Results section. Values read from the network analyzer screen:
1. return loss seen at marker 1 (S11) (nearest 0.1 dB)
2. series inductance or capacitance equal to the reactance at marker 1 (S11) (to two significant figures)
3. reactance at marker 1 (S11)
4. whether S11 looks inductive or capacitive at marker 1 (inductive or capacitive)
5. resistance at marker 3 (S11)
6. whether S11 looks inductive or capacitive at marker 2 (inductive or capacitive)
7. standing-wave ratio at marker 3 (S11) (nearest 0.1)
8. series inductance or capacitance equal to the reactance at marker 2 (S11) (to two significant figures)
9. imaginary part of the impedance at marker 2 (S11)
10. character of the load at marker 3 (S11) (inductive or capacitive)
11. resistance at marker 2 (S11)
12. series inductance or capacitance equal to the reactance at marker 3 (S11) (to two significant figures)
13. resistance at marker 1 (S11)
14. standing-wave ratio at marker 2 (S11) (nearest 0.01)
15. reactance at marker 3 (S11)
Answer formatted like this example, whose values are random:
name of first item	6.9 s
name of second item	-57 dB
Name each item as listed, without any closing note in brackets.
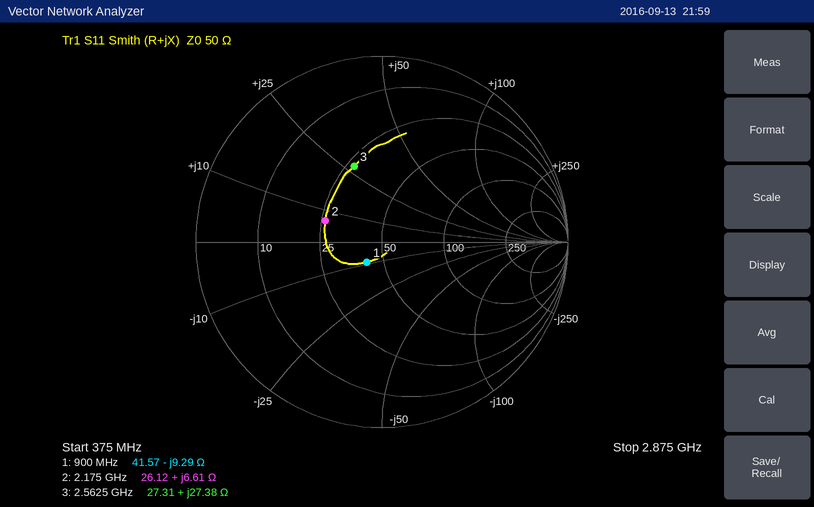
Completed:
return loss seen at marker 1 (S11)	17.3 dB
series inductance or capacitance equal to the reactance at marker 1 (S11)	19 pF
reactance at marker 1	-9.29 Ω
whether S11 looks inductive or capacitive at marker 1	capacitive
resistance at marker 3	27.31 Ω
whether S11 looks inductive or capacitive at marker 2	inductive
standing-wave ratio at marker 3 (S11)	2.5
series inductance or capacitance equal to the reactance at marker 2 (S11)	480 pH
imaginary part of the impedance at marker 2	+6.61 Ω
character of the load at marker 3 (S11)	inductive
resistance at marker 2	26.12 Ω
series inductance or capacitance equal to the reactance at marker 3 (S11)	1.7 nH
resistance at marker 1	41.57 Ω
standing-wave ratio at marker 2 (S11)	1.96
reactance at marker 3	+27.38 Ω
